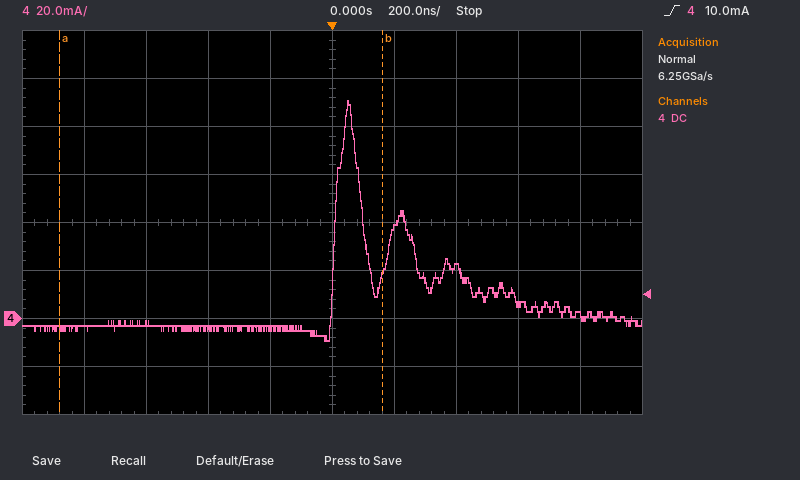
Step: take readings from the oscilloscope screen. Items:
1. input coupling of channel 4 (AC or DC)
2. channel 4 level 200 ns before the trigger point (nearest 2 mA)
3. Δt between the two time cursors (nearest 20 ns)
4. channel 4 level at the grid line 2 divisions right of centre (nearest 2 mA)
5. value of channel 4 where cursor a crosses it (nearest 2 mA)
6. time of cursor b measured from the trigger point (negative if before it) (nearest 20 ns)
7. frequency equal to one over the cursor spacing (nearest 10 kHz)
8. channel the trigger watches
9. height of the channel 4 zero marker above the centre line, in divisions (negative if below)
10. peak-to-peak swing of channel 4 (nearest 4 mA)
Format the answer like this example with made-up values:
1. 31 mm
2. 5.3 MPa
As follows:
1. DC
2. -4 mA
3. 1.04 µs
4. 22 mA
5. -4 mA
6. +160 ns
7. 960 kHz
8. channel 4
9. -2.0 div
10. 100 mA
